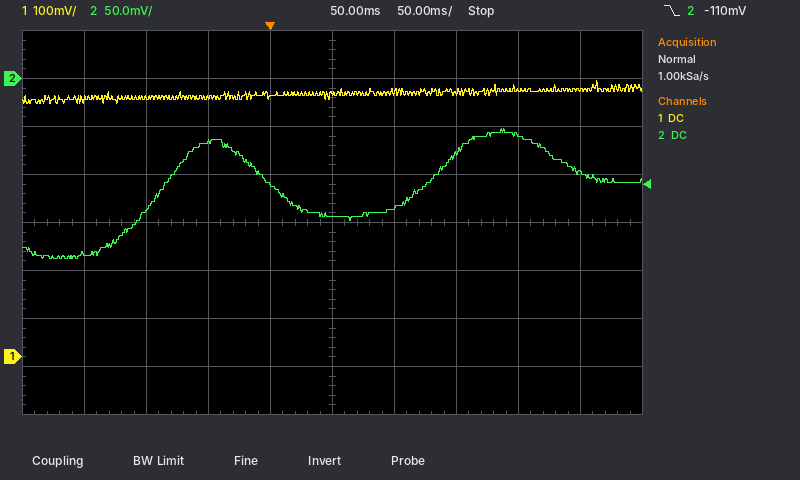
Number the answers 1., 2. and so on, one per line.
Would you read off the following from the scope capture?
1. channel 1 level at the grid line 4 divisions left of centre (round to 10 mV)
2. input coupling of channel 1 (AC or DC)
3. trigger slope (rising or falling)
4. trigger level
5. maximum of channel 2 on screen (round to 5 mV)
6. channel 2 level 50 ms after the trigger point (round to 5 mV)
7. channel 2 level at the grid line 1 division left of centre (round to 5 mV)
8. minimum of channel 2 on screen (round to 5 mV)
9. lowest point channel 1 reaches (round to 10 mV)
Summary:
1. 540 mV
2. DC
3. falling
4. -110 mV
5. -50 mV
6. -145 mV
7. -110 mV
8. -190 mV
9. 530 mV
